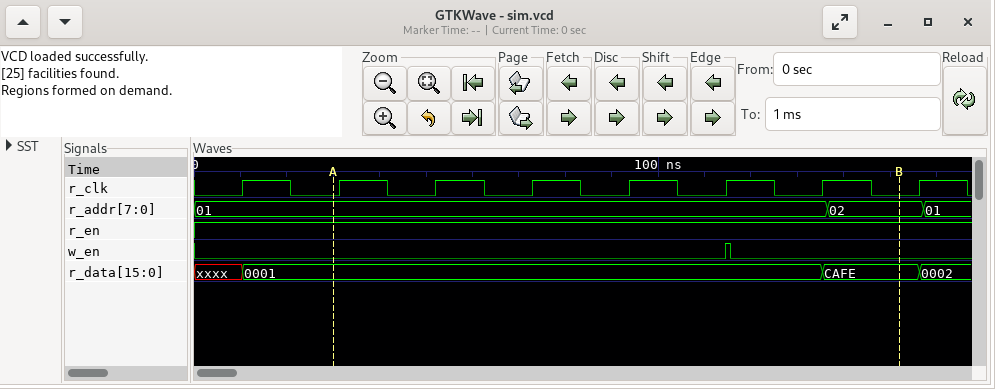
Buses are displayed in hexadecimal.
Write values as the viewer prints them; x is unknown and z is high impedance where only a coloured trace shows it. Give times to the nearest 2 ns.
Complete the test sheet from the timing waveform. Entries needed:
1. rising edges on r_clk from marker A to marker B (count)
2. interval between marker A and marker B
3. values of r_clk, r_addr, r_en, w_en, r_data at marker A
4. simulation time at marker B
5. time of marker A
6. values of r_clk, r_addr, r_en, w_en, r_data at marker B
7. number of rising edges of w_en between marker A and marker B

6
122 ns
r_clk=0, r_addr=01, r_en=1, w_en=0, r_data=0001
152 ns
30 ns
r_clk=0, r_addr=02, r_en=1, w_en=0, r_data=CAFE
1
